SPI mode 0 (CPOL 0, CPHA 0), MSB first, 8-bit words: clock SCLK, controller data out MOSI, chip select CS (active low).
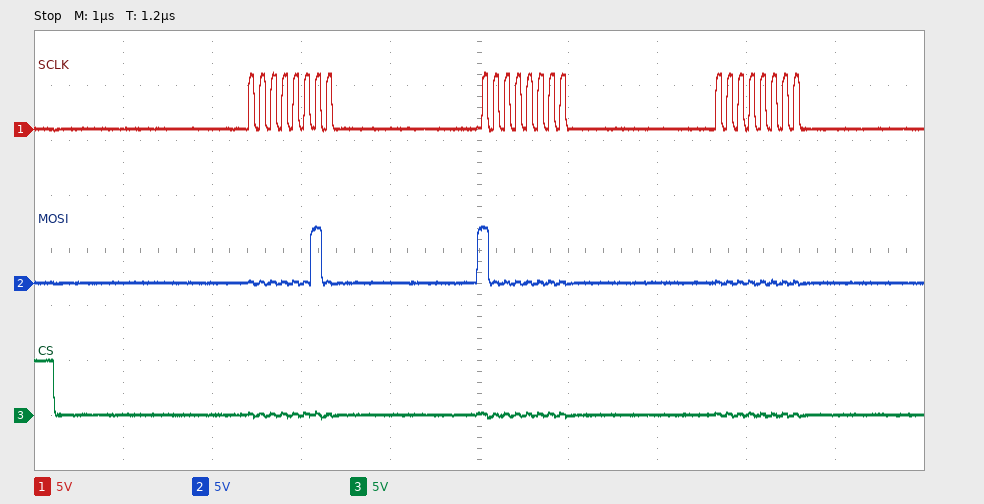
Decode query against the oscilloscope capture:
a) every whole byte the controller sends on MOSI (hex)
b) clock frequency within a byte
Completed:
02 80 00
8 MHz
